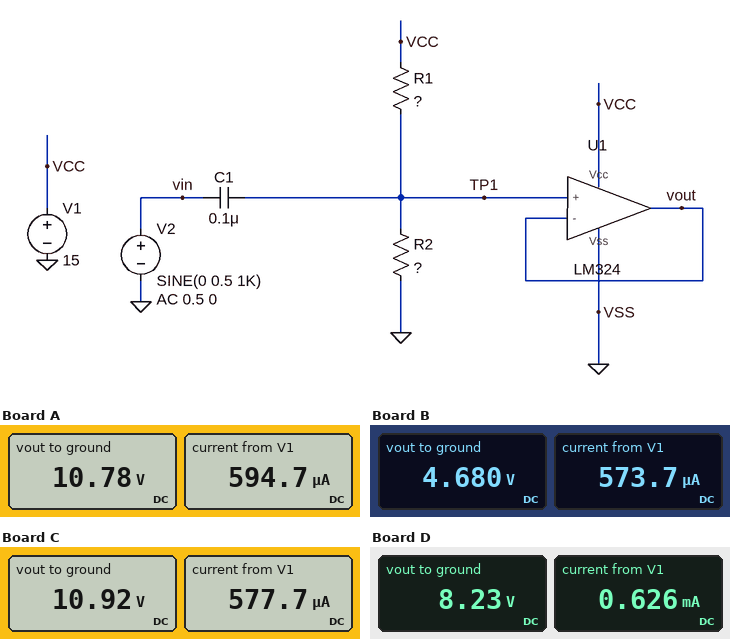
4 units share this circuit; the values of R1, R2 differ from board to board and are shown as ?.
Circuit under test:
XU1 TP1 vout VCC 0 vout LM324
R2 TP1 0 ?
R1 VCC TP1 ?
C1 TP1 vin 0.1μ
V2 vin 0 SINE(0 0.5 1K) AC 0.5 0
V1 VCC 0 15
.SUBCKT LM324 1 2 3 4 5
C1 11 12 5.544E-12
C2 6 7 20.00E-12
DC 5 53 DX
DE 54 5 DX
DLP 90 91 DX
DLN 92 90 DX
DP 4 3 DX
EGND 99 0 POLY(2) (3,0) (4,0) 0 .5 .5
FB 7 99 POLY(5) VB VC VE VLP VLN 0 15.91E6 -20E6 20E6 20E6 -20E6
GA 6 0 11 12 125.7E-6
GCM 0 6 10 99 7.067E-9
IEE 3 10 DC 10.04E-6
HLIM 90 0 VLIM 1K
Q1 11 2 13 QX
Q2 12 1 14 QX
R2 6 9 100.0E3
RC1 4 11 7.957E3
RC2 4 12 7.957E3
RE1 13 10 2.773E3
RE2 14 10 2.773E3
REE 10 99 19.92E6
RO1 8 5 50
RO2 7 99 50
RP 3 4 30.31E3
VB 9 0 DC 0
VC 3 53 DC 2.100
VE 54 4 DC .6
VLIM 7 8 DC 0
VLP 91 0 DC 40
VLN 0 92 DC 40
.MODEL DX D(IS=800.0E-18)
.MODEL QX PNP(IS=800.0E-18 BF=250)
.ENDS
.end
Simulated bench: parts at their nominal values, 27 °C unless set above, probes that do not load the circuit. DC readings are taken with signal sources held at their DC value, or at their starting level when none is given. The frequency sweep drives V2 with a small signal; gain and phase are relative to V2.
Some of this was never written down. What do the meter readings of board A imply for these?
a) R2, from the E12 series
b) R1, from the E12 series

120 kΩ
47 kΩ
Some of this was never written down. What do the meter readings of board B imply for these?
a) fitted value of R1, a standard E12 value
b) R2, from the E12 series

150 kΩ
68 kΩ
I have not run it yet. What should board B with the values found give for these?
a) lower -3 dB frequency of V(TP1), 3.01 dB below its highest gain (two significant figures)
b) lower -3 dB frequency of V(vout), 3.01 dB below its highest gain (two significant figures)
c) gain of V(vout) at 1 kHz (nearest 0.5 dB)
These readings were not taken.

34 Hz
34 Hz
0 dB
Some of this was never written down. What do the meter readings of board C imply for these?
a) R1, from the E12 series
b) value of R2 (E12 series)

56 kΩ
150 kΩ
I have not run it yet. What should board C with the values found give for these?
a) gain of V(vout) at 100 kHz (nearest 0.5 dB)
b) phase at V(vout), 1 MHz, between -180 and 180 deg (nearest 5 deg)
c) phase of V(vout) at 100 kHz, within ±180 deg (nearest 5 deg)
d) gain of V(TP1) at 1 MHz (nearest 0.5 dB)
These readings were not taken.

0 dB
-65 deg
-5 deg
0 dB
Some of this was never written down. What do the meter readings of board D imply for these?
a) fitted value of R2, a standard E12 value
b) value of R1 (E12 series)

68 kΩ
56 kΩ
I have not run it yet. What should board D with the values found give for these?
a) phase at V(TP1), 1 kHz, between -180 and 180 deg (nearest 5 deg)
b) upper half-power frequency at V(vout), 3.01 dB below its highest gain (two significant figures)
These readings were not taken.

5 deg
1.4 MHz
